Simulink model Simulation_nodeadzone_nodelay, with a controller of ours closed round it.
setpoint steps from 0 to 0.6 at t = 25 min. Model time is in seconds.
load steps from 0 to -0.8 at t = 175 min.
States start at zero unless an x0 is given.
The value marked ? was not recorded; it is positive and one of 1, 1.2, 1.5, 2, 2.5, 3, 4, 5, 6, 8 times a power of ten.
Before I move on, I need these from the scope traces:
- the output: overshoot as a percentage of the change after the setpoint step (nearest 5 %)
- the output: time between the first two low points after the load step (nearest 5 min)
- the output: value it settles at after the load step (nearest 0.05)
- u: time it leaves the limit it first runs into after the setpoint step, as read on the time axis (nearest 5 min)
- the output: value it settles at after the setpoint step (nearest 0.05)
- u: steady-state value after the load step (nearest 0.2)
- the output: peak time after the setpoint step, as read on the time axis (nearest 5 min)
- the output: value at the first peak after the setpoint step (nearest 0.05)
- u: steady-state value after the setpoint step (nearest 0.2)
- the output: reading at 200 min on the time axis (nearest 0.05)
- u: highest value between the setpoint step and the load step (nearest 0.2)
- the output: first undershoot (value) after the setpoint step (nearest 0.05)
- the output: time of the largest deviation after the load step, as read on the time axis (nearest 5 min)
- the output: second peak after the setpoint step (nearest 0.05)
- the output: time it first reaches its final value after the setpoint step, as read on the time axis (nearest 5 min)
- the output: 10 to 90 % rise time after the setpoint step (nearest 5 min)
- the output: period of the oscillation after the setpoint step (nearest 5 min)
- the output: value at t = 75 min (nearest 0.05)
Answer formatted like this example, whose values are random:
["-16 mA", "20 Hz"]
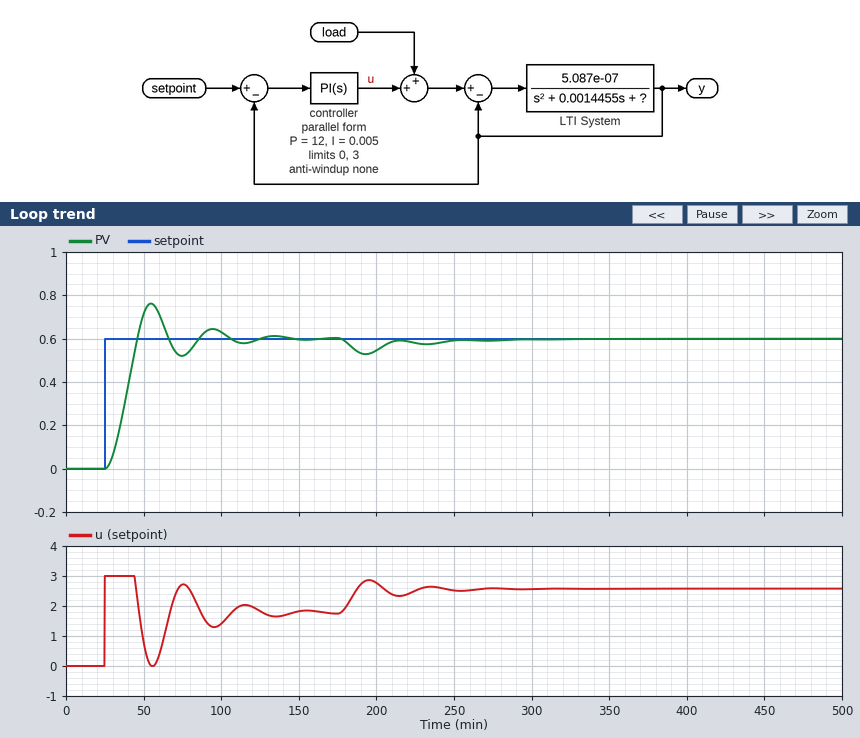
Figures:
["25 %", "40 min", "0.60", "45 min", "0.60", "2.6", "55 min", "0.75", "1.8", "0.55", "3.0", "0.50", "195 min", "0.65", "45 min", "15 min", "40 min", "0.50"]
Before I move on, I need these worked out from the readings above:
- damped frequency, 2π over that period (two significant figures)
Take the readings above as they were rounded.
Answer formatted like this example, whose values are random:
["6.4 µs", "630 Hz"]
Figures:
["0.16 rad/min"]
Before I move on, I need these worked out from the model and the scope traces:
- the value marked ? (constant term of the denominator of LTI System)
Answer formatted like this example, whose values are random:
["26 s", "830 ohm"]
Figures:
["1e-06"]
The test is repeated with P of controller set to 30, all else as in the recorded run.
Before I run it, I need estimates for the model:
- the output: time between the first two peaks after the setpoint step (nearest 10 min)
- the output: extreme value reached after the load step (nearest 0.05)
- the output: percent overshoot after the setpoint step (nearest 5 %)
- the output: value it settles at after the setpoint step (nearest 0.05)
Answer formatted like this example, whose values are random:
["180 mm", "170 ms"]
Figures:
["30 min", "0.55", "20 %", "0.60"]
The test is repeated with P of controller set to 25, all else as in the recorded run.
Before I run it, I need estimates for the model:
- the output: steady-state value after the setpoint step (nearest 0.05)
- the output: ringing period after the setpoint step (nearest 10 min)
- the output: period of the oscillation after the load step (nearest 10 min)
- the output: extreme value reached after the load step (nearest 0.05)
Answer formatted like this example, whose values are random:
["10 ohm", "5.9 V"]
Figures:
["0.60", "30 min", "30 min", "0.55"]
